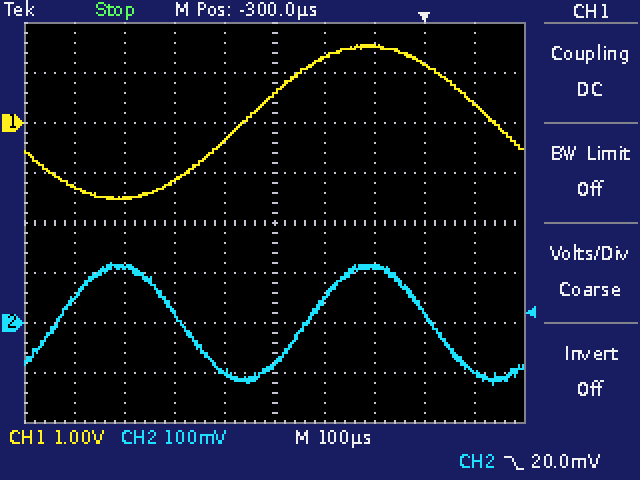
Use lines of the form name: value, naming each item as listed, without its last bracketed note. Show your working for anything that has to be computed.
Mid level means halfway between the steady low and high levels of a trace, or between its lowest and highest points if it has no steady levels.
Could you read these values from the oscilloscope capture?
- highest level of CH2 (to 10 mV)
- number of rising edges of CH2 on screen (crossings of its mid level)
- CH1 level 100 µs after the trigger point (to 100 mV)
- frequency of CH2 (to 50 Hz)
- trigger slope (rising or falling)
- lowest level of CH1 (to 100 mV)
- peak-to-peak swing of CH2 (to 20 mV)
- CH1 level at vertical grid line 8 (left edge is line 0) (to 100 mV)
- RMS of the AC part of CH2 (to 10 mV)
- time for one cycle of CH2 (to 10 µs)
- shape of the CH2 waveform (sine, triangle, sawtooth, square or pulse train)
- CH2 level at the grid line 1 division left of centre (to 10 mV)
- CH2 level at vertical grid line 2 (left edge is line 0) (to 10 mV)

highest level of CH2: 120 mV
number of rising edges of CH2 on screen: 2
CH1 level 100 µs after the trigger point: 400 mV
frequency of CH2: 1 / 500 µs ≈ 2.00 kHz
trigger slope: falling
lowest level of CH1: -1.5 V
peak-to-peak swing of CH2: 240 mV
CH1 level at vertical grid line 8 (left edge is line 0): 1.2 V
RMS of the AC part of CH2: 240 mV / (2√2) ≈ 84.9 mV, so 80 mV to the nearest 10 mV
time for one cycle of CH2: 500 µs
shape of the CH2 waveform: sine
CH2 level at the grid line 1 division left of centre: -100 mV
CH2 level at vertical grid line 2 (left edge is line 0): 110 mV
